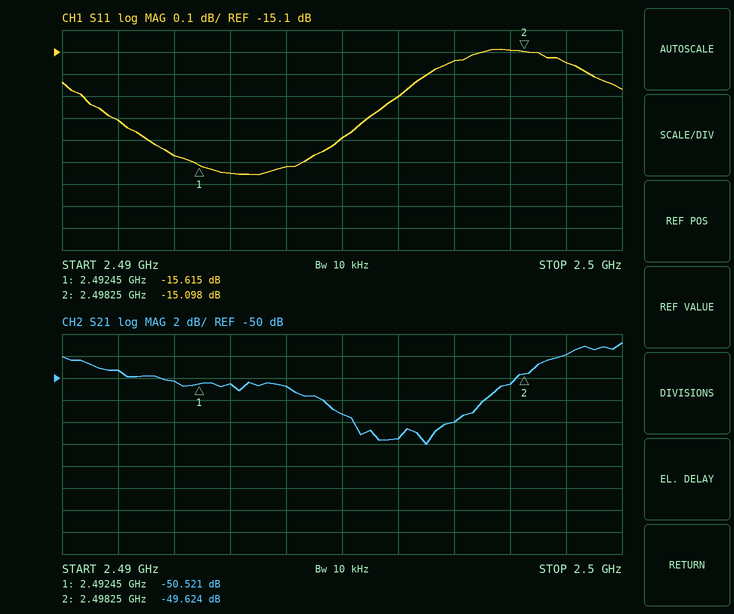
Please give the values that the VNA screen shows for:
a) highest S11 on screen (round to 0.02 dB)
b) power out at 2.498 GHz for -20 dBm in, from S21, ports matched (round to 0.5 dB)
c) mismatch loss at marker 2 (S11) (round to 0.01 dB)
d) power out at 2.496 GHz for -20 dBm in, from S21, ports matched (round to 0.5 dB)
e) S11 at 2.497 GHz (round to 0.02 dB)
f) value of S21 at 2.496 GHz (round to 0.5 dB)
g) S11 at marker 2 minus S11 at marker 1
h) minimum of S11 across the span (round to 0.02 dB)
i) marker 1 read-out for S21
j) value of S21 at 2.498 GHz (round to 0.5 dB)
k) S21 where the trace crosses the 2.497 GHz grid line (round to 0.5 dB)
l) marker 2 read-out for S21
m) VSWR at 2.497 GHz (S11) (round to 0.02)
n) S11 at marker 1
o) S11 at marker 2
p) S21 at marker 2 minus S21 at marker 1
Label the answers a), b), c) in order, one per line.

a) -15.08 dB
b) -70.5 dBm
c) 0.14 dB
d) -75.5 dBm
e) -15.14 dB
f) -55.5 dB
g) 0.517 dB
h) -15.66 dB
i) -50.521 dB
j) -50.5 dB
k) -54.0 dB
l) -49.624 dB
m) 1.42
n) -15.615 dB
o) -15.098 dB
p) 0.897 dB
